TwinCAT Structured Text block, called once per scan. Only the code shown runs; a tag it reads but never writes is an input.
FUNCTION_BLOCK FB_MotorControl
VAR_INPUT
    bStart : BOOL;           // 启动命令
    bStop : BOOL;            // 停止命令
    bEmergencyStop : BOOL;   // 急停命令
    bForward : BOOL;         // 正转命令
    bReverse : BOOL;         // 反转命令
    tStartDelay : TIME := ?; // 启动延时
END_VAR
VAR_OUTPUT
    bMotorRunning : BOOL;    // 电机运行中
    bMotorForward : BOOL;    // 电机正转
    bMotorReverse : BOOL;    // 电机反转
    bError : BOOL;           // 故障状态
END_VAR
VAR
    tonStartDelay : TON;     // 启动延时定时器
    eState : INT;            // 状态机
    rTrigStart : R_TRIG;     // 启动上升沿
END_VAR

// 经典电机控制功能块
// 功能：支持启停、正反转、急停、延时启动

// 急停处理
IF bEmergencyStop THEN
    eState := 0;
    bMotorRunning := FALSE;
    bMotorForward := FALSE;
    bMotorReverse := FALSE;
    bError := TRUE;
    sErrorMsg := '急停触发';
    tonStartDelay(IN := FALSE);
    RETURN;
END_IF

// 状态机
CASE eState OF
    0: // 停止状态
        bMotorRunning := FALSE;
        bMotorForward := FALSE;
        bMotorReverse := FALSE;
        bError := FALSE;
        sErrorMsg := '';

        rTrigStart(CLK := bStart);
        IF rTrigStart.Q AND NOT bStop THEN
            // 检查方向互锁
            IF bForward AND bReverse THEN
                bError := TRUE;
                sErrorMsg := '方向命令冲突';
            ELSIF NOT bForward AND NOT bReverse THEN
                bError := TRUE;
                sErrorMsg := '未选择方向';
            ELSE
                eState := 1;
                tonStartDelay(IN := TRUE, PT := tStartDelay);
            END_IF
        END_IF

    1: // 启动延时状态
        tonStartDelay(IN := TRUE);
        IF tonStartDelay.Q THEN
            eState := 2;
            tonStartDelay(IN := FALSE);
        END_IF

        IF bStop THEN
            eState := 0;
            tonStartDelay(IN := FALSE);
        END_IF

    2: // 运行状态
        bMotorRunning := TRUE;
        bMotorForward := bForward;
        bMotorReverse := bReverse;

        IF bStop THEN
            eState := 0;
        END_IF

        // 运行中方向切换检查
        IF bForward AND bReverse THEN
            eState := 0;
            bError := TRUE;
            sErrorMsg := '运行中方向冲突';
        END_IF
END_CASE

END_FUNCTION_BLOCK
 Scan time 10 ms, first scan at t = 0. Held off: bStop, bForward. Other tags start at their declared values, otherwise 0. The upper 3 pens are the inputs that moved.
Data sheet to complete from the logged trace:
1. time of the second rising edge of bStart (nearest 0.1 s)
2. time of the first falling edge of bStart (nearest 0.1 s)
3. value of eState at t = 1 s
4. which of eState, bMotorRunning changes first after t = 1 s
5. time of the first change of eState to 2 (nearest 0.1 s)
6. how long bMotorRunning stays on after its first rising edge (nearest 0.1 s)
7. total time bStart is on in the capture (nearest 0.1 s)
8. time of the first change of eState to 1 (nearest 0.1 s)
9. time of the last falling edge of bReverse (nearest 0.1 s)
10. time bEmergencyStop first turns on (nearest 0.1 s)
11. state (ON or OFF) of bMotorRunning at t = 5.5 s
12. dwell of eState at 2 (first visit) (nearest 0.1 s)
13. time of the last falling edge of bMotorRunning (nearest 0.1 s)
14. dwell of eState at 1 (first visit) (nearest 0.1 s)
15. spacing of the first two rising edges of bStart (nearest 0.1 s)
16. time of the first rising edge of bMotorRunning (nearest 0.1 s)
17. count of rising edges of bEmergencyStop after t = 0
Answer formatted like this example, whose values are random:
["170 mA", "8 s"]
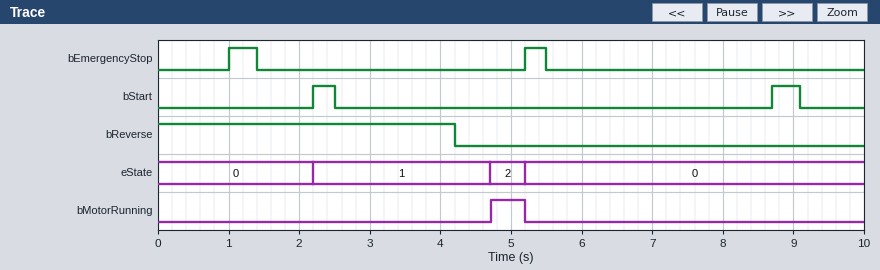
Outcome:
["8.7 s", "2.5 s", "0", "eState", "4.7 s", "0.5 s", "0.7 s", "2.2 s", "4.2 s", "1.0 s", "OFF", "0.5 s", "5.2 s", "2.5 s", "6.5 s", "4.7 s", "2"]
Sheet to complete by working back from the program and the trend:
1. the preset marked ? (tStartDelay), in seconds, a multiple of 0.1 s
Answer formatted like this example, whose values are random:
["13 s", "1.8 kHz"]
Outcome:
["2.5 s"]
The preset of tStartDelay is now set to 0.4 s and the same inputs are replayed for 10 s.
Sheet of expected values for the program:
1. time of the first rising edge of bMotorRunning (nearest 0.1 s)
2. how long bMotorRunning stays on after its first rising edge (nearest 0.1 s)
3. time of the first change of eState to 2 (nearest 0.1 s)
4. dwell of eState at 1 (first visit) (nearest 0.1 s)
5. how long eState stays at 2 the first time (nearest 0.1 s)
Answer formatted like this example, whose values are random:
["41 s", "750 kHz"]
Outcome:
["2.6 s", "2.6 s", "2.6 s", "0.4 s", "2.6 s"]
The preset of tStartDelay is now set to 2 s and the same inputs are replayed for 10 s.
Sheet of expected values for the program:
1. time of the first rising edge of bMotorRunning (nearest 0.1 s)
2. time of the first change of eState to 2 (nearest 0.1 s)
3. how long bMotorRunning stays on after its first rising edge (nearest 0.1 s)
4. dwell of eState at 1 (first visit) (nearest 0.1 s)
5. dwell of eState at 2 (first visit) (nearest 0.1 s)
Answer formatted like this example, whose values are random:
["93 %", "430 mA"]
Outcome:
["4.2 s", "4.2 s", "1.0 s", "2.0 s", "1.0 s"]
